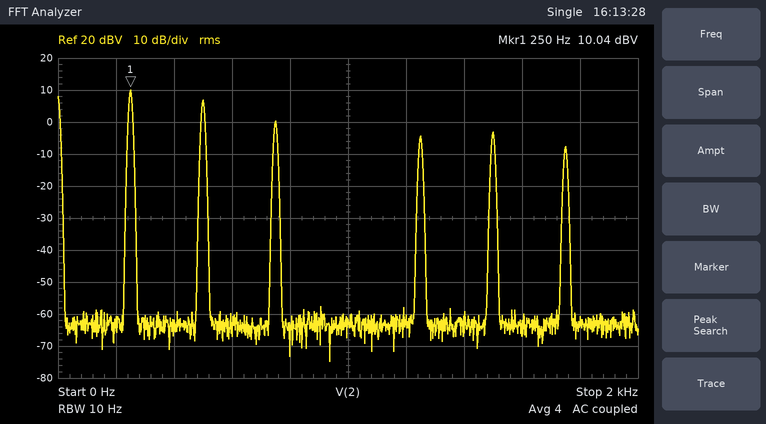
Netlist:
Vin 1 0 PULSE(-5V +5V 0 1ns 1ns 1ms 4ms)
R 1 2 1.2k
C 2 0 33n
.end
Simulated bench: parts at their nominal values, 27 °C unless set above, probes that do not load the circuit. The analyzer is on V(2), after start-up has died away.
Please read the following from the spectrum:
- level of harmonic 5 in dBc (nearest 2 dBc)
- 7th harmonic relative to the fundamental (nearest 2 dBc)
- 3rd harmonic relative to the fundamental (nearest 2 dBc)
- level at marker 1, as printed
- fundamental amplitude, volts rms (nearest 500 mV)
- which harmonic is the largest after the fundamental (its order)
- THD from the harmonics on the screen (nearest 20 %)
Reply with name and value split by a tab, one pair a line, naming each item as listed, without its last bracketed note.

level of harmonic 5 in dBc	-14 dBc
7th harmonic relative to the fundamental	-18 dBc
3rd harmonic relative to the fundamental	-10 dBc
level at marker 1, as printed	10.04 dBV
fundamental amplitude, volts rms	3.0 V
which harmonic is the largest after the fundamental	2
THD from the harmonics on the screen	80 %
